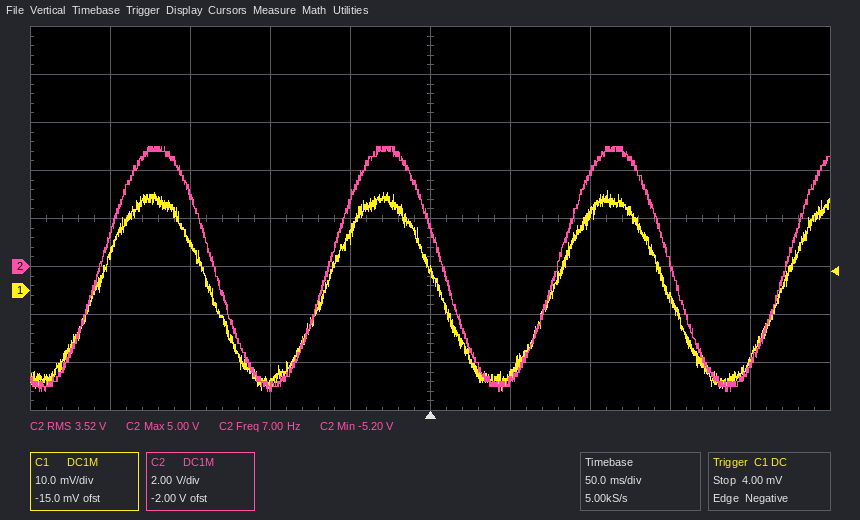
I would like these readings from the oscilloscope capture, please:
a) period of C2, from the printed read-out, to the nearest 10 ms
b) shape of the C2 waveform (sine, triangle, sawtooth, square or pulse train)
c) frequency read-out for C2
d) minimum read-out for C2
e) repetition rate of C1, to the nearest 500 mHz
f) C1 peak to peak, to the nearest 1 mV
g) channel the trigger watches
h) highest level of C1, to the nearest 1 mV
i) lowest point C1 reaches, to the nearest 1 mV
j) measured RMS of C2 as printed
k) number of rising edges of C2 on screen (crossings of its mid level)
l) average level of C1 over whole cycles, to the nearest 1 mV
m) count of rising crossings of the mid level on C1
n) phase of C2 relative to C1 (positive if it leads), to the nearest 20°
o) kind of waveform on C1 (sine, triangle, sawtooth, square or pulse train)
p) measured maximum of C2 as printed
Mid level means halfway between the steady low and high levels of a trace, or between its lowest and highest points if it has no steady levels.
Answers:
140 ms
sine
7.00 Hz
-5.20 V
7.0 Hz
42 mV
C1
21 mV
-21 mV
3.52 V
4
0 mV
4
0°
sine
5.00 V
